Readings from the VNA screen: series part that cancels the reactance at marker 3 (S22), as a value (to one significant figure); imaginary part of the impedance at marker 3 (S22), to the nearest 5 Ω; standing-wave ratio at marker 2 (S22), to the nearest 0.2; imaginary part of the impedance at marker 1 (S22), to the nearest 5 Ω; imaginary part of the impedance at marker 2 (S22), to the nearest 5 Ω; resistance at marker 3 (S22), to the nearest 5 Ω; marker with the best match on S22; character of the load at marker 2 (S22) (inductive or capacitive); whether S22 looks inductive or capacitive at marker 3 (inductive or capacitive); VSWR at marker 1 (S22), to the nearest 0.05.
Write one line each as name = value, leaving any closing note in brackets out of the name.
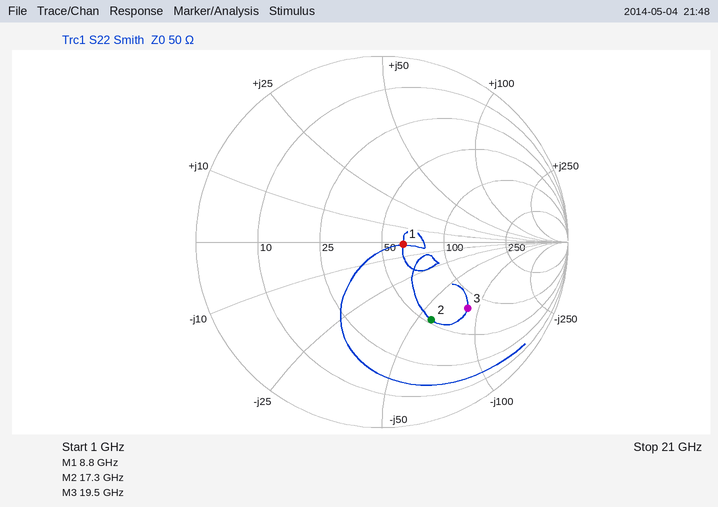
series part that cancels the reactance at marker 3 (S22), as a value = 700 pH
imaginary part of the impedance at marker 3 (S22), to the nearest 5 Ω = -85 Ω
standing-wave ratio at marker 2 (S22), to the nearest 0.2 = 3.0
imaginary part of the impedance at marker 1 (S22), to the nearest 5 Ω = 0 Ω
imaginary part of the impedance at marker 2 (S22), to the nearest 5 Ω = -60 Ω
resistance at marker 3 (S22), to the nearest 5 Ω = 80 Ω
marker with the best match on S22 = marker 1
character of the load at marker 2 (S22) = capacitive
whether S22 looks inductive or capacitive at marker 3 = capacitive
VSWR at marker 1 (S22), to the nearest 0.05 = 1.25
